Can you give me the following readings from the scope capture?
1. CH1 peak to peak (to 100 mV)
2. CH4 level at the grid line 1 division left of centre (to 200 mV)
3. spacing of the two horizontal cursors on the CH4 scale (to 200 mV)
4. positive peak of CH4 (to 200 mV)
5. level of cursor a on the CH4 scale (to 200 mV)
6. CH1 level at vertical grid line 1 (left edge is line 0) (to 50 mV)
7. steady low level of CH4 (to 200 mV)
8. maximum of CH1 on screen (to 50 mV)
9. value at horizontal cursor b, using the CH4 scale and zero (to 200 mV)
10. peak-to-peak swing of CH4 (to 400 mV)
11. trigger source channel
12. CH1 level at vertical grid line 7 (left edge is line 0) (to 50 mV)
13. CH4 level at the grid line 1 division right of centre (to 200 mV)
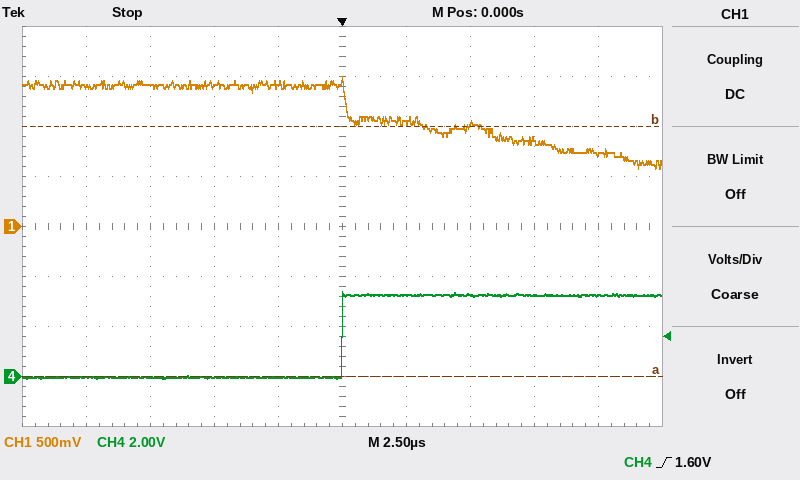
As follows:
900 mV
0.0 V
10.0 V
3.4 V
0.0 V
1.40 V
0.0 V
1.50 V
10.0 V
3.6 V
CH4
1.00 V
3.2 V
